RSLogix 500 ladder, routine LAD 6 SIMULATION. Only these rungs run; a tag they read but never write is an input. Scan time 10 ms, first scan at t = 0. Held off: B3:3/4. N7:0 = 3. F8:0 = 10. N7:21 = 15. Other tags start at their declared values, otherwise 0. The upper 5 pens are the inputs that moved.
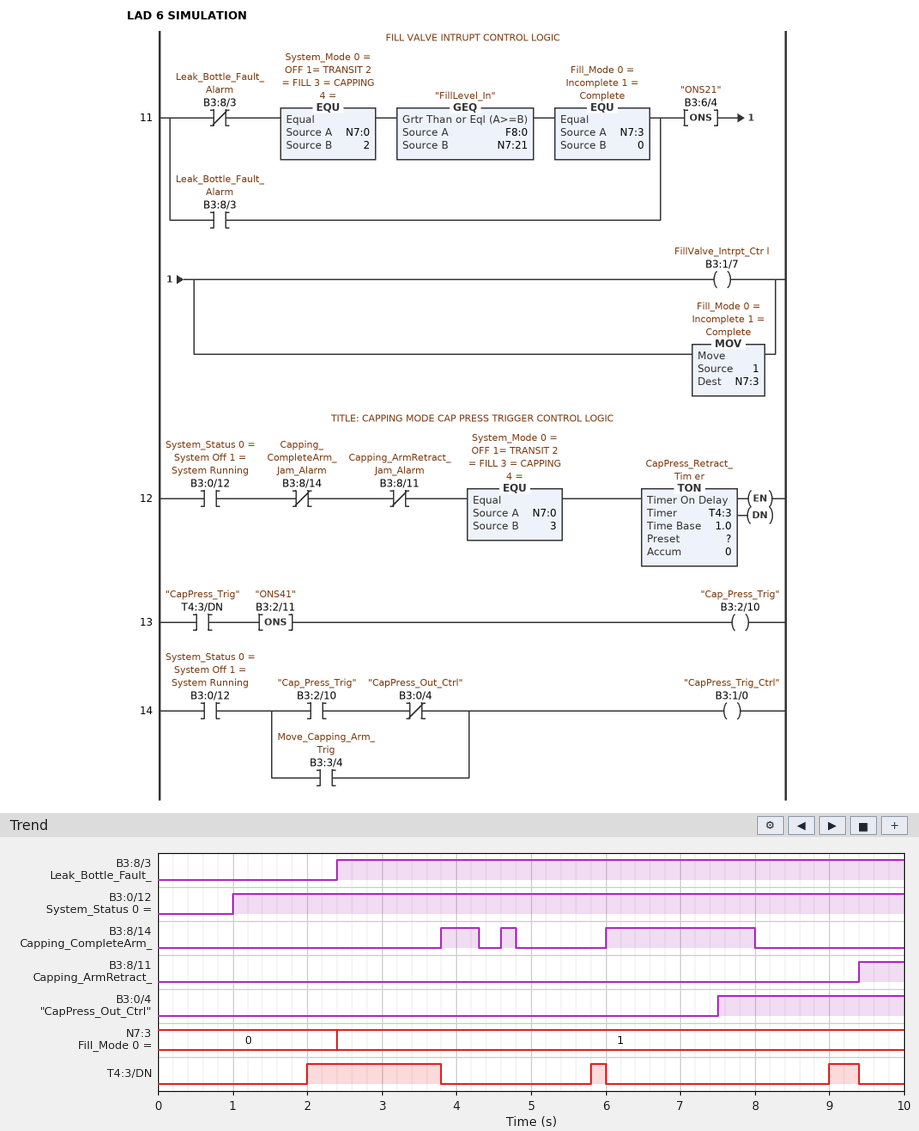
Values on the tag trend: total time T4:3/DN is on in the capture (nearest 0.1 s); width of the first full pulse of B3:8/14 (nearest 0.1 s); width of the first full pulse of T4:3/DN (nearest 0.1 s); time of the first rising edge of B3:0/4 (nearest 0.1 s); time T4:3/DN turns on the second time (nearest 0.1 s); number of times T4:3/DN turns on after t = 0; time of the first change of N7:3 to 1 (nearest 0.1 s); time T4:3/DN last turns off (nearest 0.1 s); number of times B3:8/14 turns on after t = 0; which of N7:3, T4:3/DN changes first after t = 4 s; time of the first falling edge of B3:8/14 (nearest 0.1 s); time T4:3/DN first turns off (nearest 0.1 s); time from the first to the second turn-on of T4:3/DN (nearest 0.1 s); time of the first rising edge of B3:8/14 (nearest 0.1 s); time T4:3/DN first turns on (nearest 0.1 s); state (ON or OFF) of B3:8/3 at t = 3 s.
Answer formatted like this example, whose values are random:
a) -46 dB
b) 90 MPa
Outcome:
a) 2.4 s
b) 0.5 s
c) 1.8 s
d) 7.5 s
e) 5.8 s
f) 3
g) 2.4 s
h) 9.4 s
i) 3
j) T4:3/DN
k) 4.3 s
l) 3.8 s
m) 3.8 s
n) 3.8 s
o) 2.0 s
p) ON
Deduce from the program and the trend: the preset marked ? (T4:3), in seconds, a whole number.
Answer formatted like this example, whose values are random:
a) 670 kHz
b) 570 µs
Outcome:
a) 1 s
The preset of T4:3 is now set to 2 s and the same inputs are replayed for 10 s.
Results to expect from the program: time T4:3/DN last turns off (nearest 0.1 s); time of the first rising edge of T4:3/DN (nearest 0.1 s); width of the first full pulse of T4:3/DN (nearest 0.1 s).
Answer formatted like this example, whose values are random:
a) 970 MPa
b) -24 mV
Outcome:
a) 3.8 s
b) 3.0 s
c) 0.8 s
